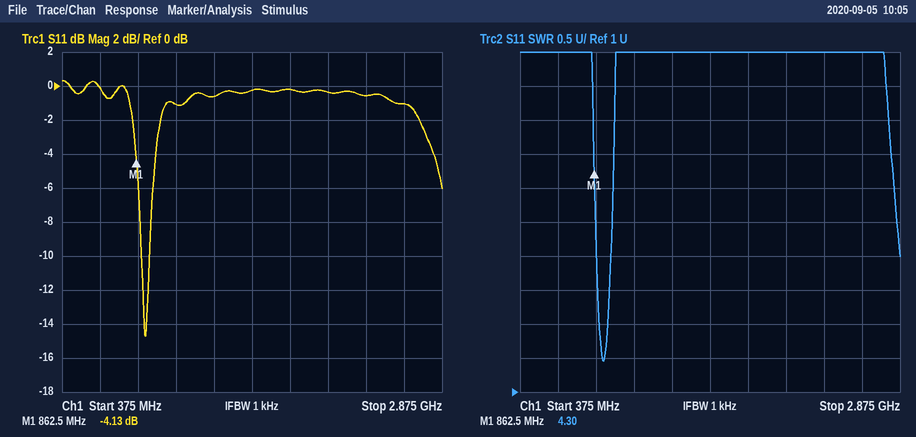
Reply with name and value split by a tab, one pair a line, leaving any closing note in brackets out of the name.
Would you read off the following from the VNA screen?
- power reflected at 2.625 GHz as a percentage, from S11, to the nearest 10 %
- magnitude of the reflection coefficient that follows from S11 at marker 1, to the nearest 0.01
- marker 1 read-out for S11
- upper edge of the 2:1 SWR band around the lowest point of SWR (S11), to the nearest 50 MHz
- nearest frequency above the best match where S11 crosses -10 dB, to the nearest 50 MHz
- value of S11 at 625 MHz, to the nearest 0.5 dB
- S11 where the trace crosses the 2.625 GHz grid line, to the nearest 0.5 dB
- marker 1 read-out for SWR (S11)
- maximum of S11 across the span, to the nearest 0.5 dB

power reflected at 2.625 GHz as a percentage, from S11, to the nearest 10 %	80 %
magnitude of the reflection coefficient that follows from S11 at marker 1, to the nearest 0.01	0.62
marker 1 read-out for S11	-4.13 dB
upper edge of the 2:1 SWR band around the lowest point of SWR (S11), to the nearest 50 MHz	950 MHz
nearest frequency above the best match where S11 crosses -10 dB, to the nearest 50 MHz	950 MHz
value of S11 at 625 MHz, to the nearest 0.5 dB	0.0 dB
S11 where the trace crosses the 2.625 GHz grid line, to the nearest 0.5 dB	-1.0 dB
marker 1 read-out for SWR	4.30
maximum of S11 across the span, to the nearest 0.5 dB	0.5 dB
